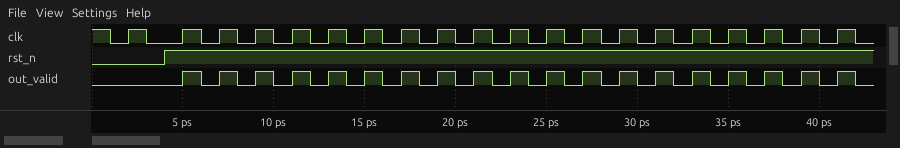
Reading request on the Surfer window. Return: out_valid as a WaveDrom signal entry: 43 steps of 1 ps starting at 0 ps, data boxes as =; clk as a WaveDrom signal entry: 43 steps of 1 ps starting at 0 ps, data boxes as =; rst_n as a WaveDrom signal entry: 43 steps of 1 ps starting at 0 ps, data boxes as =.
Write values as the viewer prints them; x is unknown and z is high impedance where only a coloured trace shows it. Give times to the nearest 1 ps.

{name: 'out_valid', wave: '0....10101010101010101010101010101010101010'}
{name: 'clk', wave: '1010.10101010101010101010101010101010101010'}
{name: 'rst_n', wave: '0...1......................................'}
